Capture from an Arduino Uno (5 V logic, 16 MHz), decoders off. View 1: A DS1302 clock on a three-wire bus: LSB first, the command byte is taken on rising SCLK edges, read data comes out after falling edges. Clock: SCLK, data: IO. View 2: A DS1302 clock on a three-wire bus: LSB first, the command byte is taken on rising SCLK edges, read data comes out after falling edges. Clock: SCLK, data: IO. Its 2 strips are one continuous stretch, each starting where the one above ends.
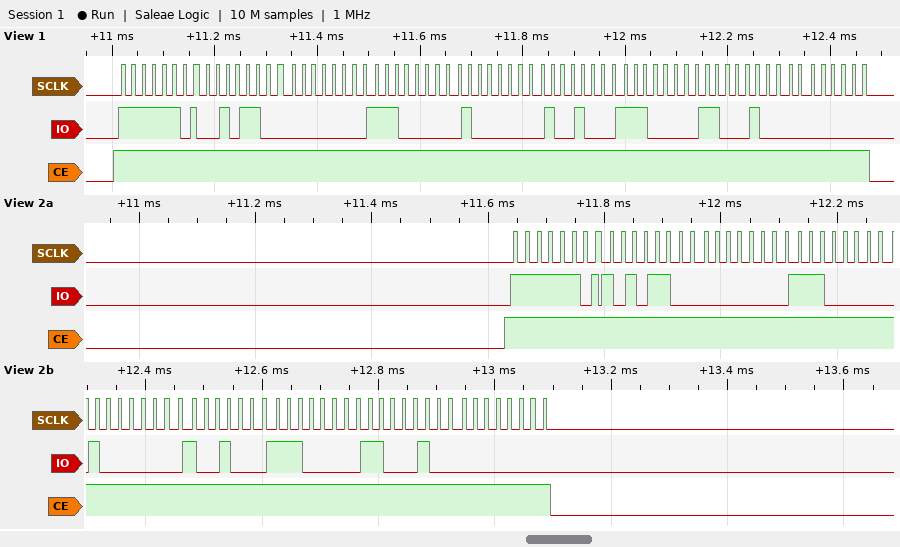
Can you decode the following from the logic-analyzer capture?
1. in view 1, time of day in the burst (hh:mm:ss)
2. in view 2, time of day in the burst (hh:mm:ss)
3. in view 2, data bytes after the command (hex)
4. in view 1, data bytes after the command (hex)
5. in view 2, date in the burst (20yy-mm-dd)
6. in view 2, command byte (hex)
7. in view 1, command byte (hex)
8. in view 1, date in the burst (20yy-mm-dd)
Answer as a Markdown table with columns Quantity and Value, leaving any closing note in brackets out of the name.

| Quantity | Value |
|---|---|
| in view 1, time of day in the burst | 07:00:34 |
| in view 2, time of day in the burst | 07:00:35 |
| in view 2, data bytes after the command | 35 00 07 02 12 07 23 00 |
| in view 1, data bytes after the command | 34 00 07 02 12 07 23 00 |
| in view 2, date in the burst | 2023-12-02 |
| in view 2, command byte | 0xBF |
| in view 1, command byte | 0xBF |
| in view 1, date in the burst | 2023-12-02 |
